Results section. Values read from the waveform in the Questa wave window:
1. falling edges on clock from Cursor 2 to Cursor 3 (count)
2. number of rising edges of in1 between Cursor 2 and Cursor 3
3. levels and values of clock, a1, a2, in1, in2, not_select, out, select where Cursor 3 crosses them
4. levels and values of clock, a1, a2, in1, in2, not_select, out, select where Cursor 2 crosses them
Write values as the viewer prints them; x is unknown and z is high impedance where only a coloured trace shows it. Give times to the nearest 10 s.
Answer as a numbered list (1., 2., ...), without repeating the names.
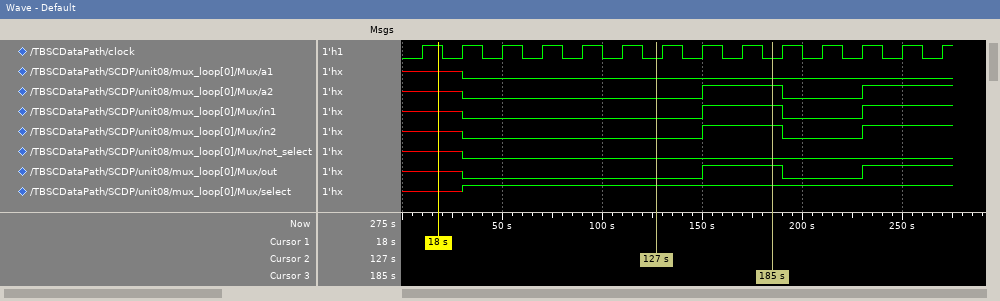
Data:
1. 3
2. 1
3. clock=0, a1=0, a2=1, in1=1, in2=1, not_select=0, out=1, select=1
4. clock=0, a1=0, a2=0, in1=0, in2=0, not_select=0, out=0, select=1
